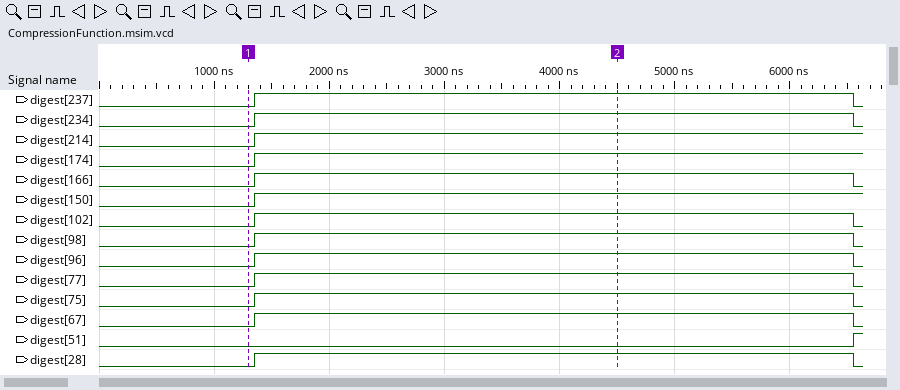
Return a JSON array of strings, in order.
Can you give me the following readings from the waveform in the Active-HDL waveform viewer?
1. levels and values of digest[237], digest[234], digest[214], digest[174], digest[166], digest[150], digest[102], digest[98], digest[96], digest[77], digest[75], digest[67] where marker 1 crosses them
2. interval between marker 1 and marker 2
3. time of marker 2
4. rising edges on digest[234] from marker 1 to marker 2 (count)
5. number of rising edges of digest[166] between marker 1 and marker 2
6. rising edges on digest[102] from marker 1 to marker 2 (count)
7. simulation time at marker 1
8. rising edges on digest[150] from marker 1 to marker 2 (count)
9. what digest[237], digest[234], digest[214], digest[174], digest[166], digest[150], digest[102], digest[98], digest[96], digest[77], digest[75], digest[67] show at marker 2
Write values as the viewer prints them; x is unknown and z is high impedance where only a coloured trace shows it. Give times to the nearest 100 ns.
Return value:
["digest[237]=0, digest[234]=0, digest[214]=0, digest[174]=0, digest[166]=0, digest[150]=0, digest[102]=0, digest[98]=0, digest[96]=0, digest[77]=0, digest[75]=0, digest[67]=0", "3200 ns", "4500 ns", "1", "1", "1", "1300 ns", "1", "digest[237]=1, digest[234]=1, digest[214]=1, digest[174]=1, digest[166]=1, digest[150]=1, digest[102]=1, digest[98]=1, digest[96]=1, digest[77]=1, digest[75]=1, digest[67]=1"]
